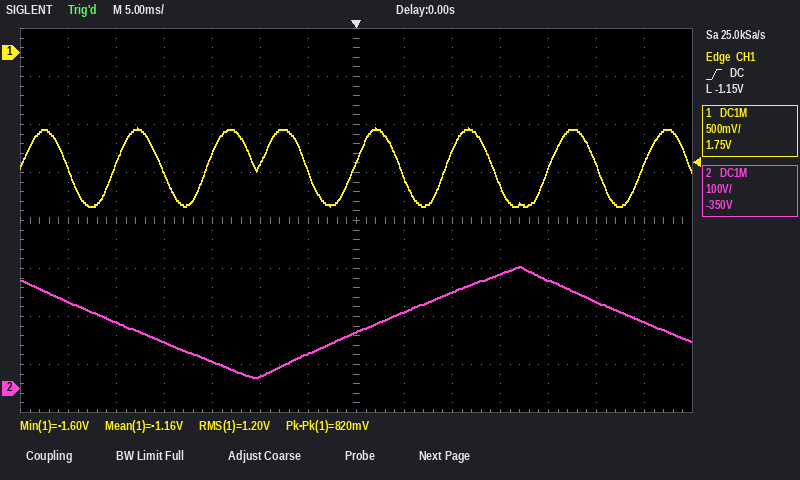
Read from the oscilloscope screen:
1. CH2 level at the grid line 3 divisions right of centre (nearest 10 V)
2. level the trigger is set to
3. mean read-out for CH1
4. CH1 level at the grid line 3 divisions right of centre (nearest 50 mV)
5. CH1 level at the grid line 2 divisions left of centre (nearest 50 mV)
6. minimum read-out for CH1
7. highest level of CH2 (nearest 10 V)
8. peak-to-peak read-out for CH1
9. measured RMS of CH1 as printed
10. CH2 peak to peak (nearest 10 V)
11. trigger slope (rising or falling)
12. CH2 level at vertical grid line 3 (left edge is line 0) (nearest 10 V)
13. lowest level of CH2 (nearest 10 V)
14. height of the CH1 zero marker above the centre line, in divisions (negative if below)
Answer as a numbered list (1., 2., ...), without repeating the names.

1. 240 V
2. -1.15 V
3. -1.16 V
4. -1.40 V
5. -1.15 V
6. -1.60 V
7. 250 V
8. 820 mV
9. 1.20 V
10. 230 V
11. rising
12. 100 V
13. 20 V
14. +3.5 div
